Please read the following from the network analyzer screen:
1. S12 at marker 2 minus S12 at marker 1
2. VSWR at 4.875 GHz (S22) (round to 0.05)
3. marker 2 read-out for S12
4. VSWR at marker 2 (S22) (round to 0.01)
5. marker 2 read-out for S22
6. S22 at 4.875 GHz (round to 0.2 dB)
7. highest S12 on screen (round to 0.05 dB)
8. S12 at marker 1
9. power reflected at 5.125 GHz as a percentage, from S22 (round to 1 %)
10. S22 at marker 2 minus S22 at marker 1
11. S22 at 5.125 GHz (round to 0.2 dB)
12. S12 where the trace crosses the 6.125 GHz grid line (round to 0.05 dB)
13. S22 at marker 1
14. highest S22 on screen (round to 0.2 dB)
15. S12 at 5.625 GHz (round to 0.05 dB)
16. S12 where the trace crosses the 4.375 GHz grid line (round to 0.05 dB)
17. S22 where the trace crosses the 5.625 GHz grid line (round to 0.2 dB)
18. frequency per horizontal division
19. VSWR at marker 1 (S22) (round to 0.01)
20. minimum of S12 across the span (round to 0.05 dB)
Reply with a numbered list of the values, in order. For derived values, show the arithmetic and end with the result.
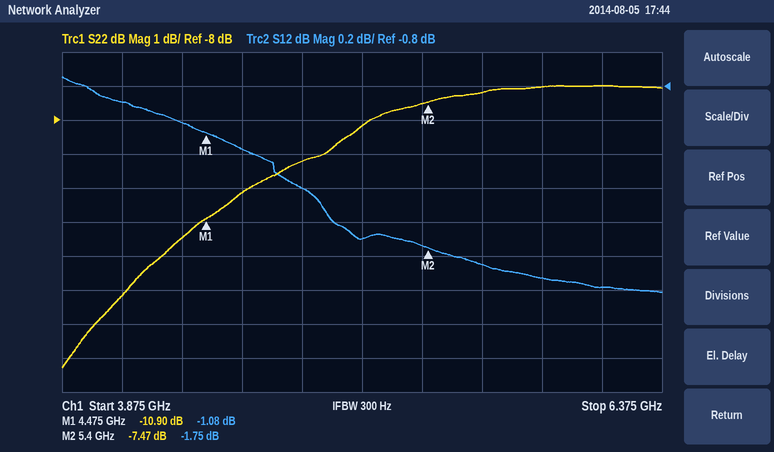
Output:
1. -1.75 − (-1.08) = -0.67 dB
2. |Γ| = 10^(-9.2/20) = 0.3467; VSWR = (1 + 0.3467)/(1 − 0.3467) ≈ 2.06, so 2.05 to the nearest 0.05
3. -1.75 dB
4. (1 + 0.4232)/(1 − 0.4232) ≈ 2.47
5. -7.47 dB
6. -9.2 dB
7. -0.75 dB
8. -1.08 dB
9. 10^(-8.2/10) ≈ 15 %
10. -7.47 − (-10.9) = 3.43 dB
11. -8.2 dB
12. -2.00 dB
13. -10.90 dB
14. -7.0 dB
15. -1.85 dB
16. -1.00 dB
17. -7.2 dB
18. 250 MHz
19. (1 + 0.2851)/(1 − 0.2851) ≈ 1.80
20. -2.00 dB
